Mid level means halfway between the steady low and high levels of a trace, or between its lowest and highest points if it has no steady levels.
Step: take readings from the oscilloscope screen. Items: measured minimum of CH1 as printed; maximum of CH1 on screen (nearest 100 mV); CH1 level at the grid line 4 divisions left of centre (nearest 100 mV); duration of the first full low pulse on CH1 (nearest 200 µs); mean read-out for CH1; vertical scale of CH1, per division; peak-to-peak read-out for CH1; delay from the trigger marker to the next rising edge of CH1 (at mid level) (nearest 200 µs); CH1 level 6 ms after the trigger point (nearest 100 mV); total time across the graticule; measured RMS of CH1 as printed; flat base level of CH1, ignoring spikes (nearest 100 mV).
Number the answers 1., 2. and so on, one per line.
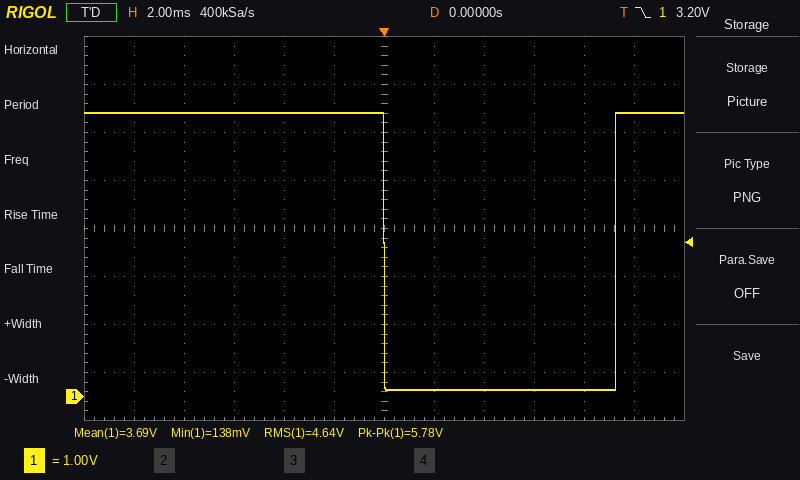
1. 138 mV
2. 5.9 V
3. 5.9 V
4. 9.2 ms
5. 3.69 V
6. 1 V
7. 5.78 V
8. 9.2 ms
9. 100 mV
10. 24 ms
11. 4.64 V
12. 100 mV
